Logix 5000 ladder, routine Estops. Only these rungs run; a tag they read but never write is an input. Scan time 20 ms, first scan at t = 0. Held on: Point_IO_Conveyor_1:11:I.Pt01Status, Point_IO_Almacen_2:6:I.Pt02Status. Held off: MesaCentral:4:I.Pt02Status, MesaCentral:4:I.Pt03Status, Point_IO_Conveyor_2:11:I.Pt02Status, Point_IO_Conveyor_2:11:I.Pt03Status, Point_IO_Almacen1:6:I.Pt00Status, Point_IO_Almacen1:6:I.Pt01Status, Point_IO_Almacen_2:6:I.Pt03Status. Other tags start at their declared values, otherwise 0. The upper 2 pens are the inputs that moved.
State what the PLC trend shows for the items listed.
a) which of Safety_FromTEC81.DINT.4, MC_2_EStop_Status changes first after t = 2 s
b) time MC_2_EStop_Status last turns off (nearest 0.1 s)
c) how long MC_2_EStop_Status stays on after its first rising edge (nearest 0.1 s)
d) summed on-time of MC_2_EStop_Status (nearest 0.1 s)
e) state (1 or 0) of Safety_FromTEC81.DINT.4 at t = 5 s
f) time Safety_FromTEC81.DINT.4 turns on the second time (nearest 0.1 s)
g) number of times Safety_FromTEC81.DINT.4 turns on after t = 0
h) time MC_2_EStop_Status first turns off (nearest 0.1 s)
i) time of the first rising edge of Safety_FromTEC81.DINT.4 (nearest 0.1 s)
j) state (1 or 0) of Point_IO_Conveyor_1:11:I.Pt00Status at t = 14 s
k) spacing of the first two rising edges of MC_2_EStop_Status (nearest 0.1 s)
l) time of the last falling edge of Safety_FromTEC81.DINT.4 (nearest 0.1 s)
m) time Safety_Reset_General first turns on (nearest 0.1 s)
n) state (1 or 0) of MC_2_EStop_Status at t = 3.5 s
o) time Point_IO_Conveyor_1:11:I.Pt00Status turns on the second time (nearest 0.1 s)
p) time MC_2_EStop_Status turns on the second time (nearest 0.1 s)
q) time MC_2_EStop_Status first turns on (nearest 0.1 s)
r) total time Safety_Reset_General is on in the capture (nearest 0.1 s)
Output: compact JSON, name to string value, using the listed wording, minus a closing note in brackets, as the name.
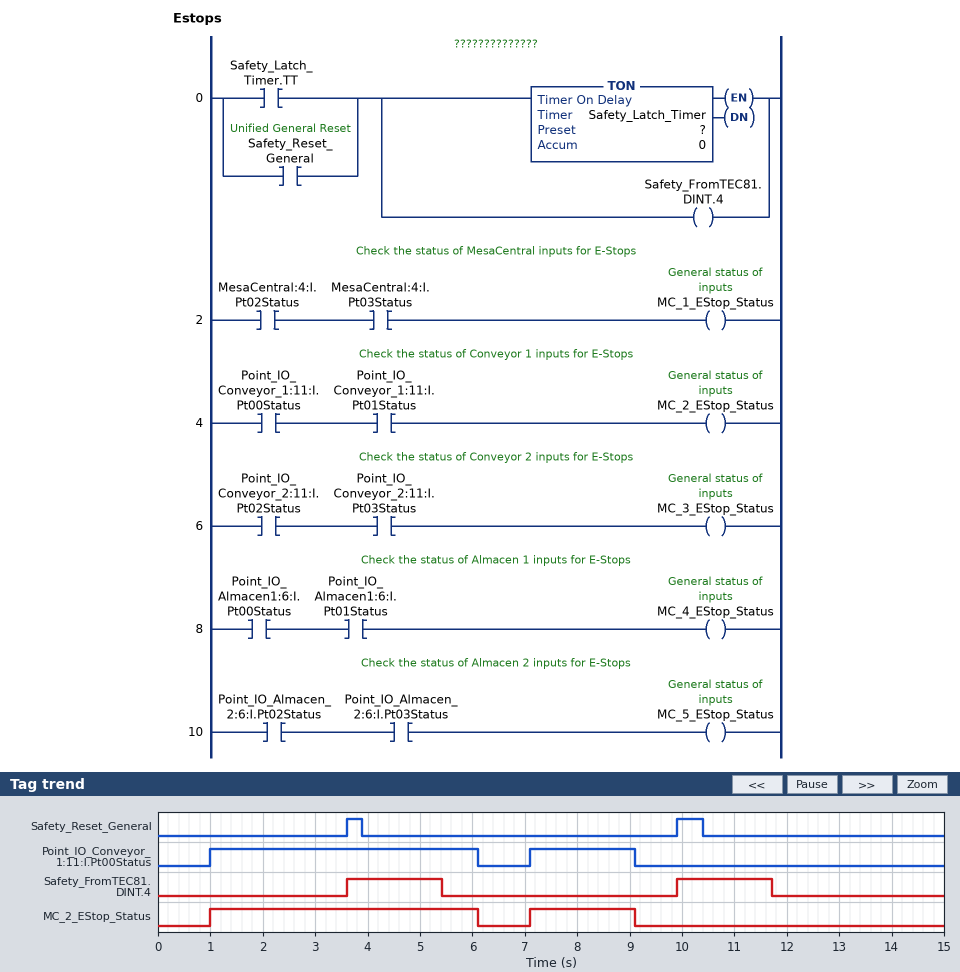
{"which of Safety_FromTEC81.DINT.4, MC_2_EStop_Status changes first after t = 2 s": "Safety_FromTEC81.DINT.4", "time MC_2_EStop_Status last turns off": "9.1 s", "how long MC_2_EStop_Status stays on after its first rising edge": "5.1 s", "summed on-time of MC_2_EStop_Status": "7.1 s", "state (1 or 0) of Safety_FromTEC81.DINT.4 at t = 5 s": "1", "time Safety_FromTEC81.DINT.4 turns on the second time": "9.9 s", "number of times Safety_FromTEC81.DINT.4 turns on after t = 0": "2", "time MC_2_EStop_Status first turns off": "6.1 s", "time of the first rising edge of Safety_FromTEC81.DINT.4": "3.6 s", "state (1 or 0) of Point_IO_Conveyor_1:11:I.Pt00Status at t = 14 s": "0", "spacing of the first two rising edges of MC_2_EStop_Status": "6.1 s", "time of the last falling edge of Safety_FromTEC81.DINT.4": "11.7 s", "time Safety_Reset_General first turns on": "3.6 s", "state (1 or 0) of MC_2_EStop_Status at t = 3.5 s": "1", "time Point_IO_Conveyor_1:11:I.Pt00Status turns on the second time": "7.1 s", "time MC_2_EStop_Status turns on the second time": "7.1 s", "time MC_2_EStop_Status first turns on": "1.0 s", "total time Safety_Reset_General is on in the capture": "0.8 s"}
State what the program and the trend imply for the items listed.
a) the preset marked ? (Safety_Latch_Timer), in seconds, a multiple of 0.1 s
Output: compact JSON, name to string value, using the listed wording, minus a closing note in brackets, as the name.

{"the preset marked ? (Safety_Latch_Timer), in seconds, a multiple of 0.1 s": "1.8 s"}
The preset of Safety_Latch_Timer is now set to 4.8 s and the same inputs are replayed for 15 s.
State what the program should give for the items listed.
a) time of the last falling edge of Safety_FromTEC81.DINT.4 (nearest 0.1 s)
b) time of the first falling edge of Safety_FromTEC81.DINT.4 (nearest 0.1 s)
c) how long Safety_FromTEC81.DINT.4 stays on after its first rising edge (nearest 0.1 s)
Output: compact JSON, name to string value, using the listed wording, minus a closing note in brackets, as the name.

{"time of the last falling edge of Safety_FromTEC81.DINT.4": "14.7 s", "time of the first falling edge of Safety_FromTEC81.DINT.4": "8.4 s", "how long Safety_FromTEC81.DINT.4 stays on after its first rising edge": "4.8 s"}
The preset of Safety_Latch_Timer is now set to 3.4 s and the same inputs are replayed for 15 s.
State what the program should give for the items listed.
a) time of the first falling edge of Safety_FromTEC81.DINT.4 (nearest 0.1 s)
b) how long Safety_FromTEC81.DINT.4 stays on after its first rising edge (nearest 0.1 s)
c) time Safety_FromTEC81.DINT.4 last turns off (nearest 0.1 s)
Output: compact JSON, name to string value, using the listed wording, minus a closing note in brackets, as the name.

{"time of the first falling edge of Safety_FromTEC81.DINT.4": "7.0 s", "how long Safety_FromTEC81.DINT.4 stays on after its first rising edge": "3.4 s", "time Safety_FromTEC81.DINT.4 last turns off": "13.3 s"}
